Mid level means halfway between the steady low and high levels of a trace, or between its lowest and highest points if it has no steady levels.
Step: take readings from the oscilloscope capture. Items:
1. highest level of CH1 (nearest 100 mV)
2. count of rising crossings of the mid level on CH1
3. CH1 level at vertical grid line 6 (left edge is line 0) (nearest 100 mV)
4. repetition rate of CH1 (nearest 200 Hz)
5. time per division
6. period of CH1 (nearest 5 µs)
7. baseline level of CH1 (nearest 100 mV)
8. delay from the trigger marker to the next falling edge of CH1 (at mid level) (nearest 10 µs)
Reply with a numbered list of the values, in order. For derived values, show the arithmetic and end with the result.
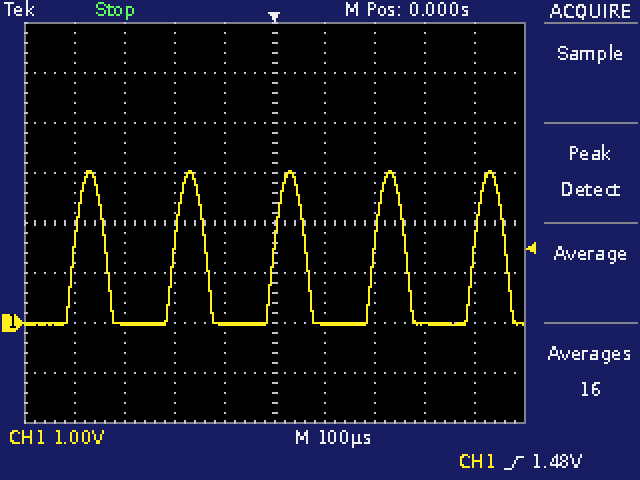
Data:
1. 3.0 V
2. 5
3. 0.0 V
4. 1 / 200 µs ≈ 5.0 kHz
5. 100 µs
6. 200 µs
7. 0.0 V
8. 60 µs
